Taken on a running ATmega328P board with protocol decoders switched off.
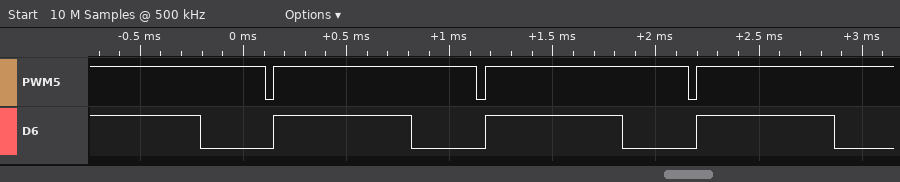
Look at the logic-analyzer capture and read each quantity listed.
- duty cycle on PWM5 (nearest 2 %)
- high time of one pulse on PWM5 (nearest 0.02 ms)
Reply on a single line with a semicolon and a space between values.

96 %; 0.98 ms
